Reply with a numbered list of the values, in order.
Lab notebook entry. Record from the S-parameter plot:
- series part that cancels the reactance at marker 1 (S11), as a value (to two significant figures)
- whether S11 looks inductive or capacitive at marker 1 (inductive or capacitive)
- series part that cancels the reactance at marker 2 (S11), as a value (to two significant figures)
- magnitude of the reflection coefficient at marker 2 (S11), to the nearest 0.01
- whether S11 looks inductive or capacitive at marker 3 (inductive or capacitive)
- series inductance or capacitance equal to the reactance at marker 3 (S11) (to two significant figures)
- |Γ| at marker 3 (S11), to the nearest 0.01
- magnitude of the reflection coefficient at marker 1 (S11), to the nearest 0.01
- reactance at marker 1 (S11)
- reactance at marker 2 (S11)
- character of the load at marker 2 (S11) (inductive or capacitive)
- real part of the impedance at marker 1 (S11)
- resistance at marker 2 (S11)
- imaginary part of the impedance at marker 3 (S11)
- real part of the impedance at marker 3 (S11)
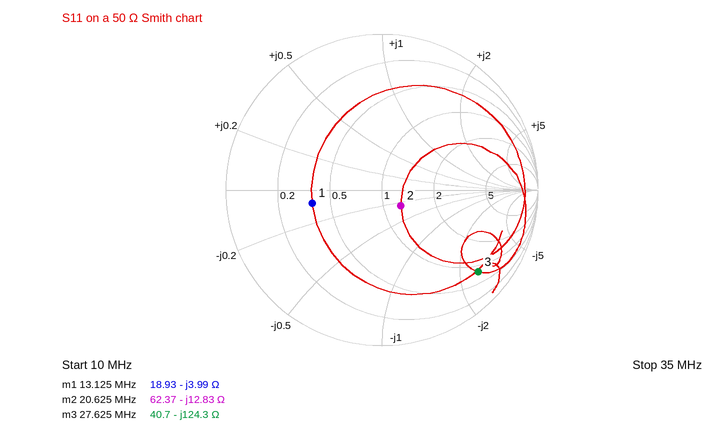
1. 48 nH
2. capacitive
3. 99 nH
4. 0.16
5. capacitive
6. 46 pF
7. 0.81
8. 0.45
9. -3.99 Ω
10. -12.83 Ω
11. capacitive
12. 18.93 Ω
13. 62.37 Ω
14. -124.3 Ω
15. 40.7 Ω
